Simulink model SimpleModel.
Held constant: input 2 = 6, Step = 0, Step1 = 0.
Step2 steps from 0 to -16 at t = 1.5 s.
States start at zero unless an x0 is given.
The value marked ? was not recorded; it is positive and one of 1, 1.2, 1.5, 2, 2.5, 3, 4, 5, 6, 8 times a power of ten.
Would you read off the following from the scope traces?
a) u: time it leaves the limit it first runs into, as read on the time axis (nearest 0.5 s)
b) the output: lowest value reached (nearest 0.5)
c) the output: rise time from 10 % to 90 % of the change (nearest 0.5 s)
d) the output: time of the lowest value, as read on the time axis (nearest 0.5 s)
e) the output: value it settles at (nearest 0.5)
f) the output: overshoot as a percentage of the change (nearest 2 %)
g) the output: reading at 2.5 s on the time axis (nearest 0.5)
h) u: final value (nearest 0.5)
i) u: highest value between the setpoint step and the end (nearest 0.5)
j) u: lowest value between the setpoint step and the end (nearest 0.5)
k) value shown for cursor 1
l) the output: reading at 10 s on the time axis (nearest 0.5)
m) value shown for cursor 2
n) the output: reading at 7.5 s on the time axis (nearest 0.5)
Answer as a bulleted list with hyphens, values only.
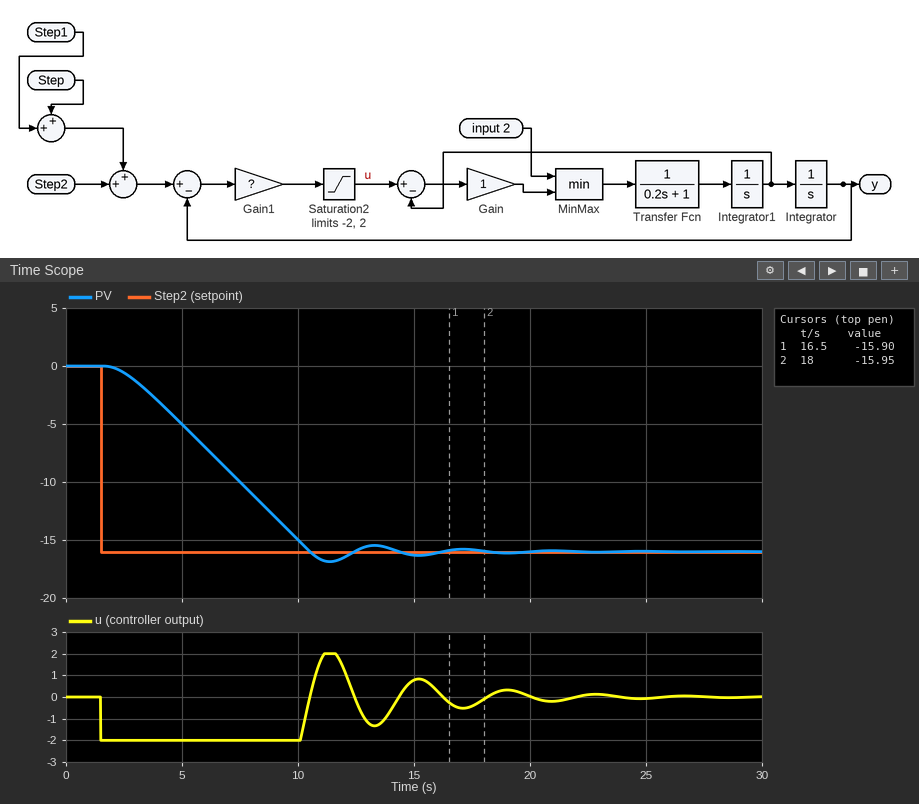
- 10.0 s
- -17.0
- 6.5 s
- 11.5 s
- -16.0
- 6 %
- -0.5
- 0.0
- 2.0
- -2.0
- -15.90
- -15.0
- -15.95
- -10.0
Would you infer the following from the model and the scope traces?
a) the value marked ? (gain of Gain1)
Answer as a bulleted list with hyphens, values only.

- 2.5
